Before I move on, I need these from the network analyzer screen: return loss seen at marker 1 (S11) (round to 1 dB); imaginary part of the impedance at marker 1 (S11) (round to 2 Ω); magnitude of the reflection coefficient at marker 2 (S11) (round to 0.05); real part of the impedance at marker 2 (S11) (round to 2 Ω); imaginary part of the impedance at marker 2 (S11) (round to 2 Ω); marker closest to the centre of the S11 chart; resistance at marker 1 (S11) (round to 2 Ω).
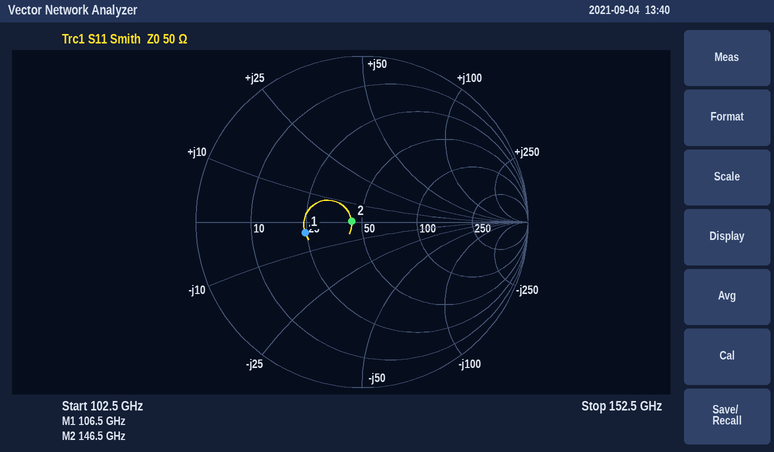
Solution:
9 dB
-4 Ω
0.05
44 Ω
0 Ω
marker 2
24 Ω
